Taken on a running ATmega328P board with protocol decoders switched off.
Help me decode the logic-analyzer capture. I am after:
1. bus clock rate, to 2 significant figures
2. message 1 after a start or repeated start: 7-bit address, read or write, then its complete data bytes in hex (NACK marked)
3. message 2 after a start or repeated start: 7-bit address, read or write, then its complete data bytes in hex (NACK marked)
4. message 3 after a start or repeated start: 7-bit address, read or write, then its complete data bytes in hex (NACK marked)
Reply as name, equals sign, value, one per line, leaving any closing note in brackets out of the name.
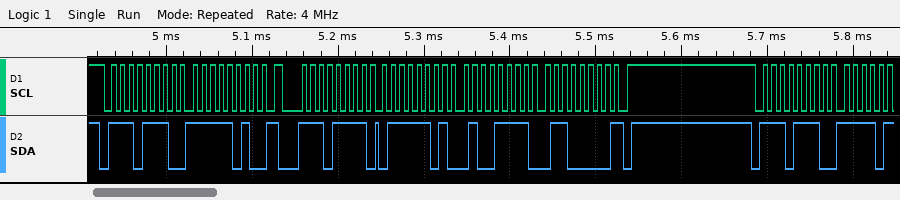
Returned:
bus clock rate, to 2 significant figures = 100 kHz
message 1 after a start or repeated start: 7-bit address, read or write, then its complete data bytes in hex = 0x77 write: FA
message 2 after a start or repeated start: 7-bit address, read or write, then its complete data bytes in hex = 0x77 read: 7D 4F 60 NACK
message 3 after a start or repeated start: 7-bit address, read or write, then its complete data bytes in hex = 0x77 write
